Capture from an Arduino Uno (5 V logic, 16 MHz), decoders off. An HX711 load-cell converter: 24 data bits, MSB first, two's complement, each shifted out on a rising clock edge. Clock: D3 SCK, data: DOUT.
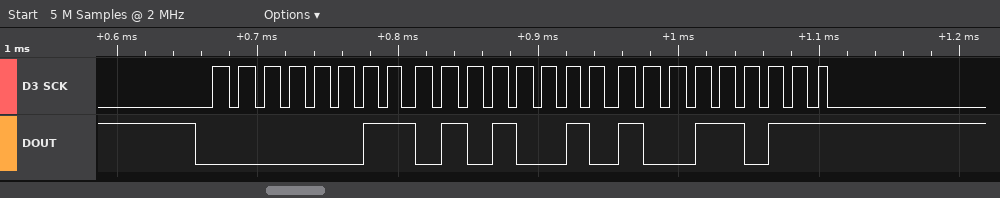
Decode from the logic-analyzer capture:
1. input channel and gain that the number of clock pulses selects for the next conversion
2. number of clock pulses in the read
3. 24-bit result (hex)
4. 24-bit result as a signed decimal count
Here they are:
channel A, gain 128
25
0x03529B
217755
